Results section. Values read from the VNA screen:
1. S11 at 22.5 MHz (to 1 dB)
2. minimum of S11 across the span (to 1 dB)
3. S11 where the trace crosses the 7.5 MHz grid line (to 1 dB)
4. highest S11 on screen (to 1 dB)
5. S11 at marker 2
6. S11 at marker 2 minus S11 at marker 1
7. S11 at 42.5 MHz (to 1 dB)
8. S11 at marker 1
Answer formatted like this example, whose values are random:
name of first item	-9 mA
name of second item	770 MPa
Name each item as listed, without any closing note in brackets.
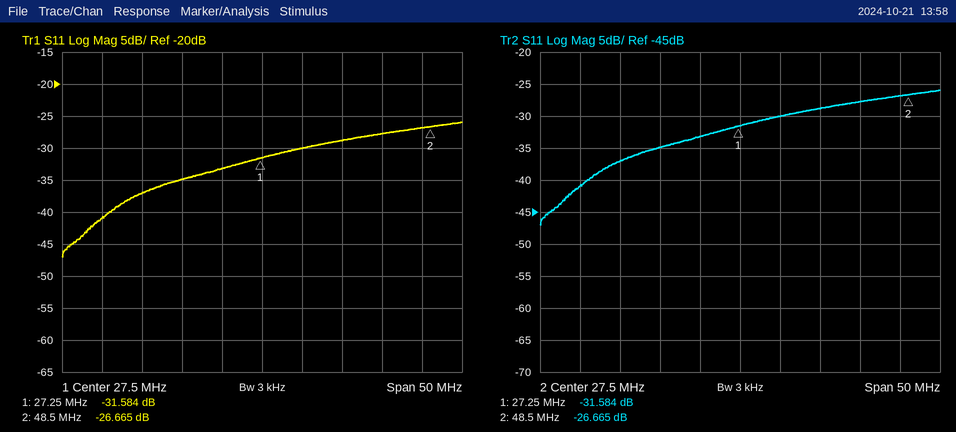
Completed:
S11 at 22.5 MHz	-33 dB
minimum of S11 across the span	-47 dB
S11 where the trace crosses the 7.5 MHz grid line	-41 dB
highest S11 on screen	-26 dB
S11 at marker 2	-26.665 dB
S11 at marker 2 minus S11 at marker 1	4.919 dB
S11 at 42.5 MHz	-28 dB
S11 at marker 1	-31.584 dB
